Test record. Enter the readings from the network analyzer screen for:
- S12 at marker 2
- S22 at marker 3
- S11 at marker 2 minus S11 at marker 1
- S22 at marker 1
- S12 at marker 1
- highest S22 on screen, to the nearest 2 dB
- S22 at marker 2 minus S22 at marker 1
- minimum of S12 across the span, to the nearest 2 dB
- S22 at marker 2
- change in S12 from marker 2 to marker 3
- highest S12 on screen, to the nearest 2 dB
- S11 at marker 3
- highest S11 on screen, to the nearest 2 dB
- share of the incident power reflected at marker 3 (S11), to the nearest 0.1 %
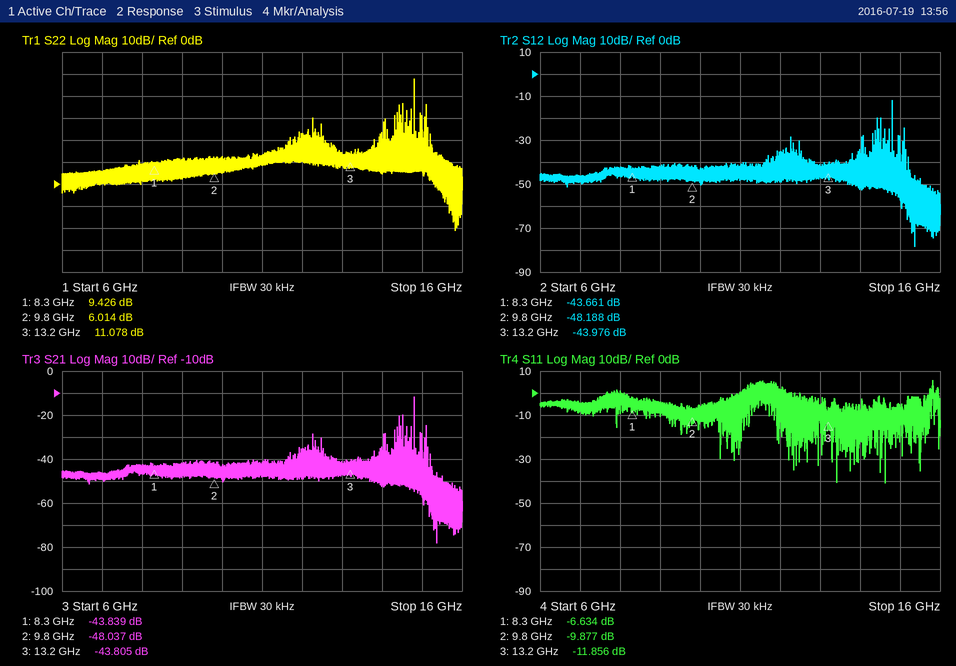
-48.188 dB
11.078 dB
-3.243 dB
9.426 dB
-43.661 dB
48 dB
-3.412 dB
-78 dB
6.014 dB
4.212 dB
-12 dB
-11.856 dB
6 dB
6.5 %
